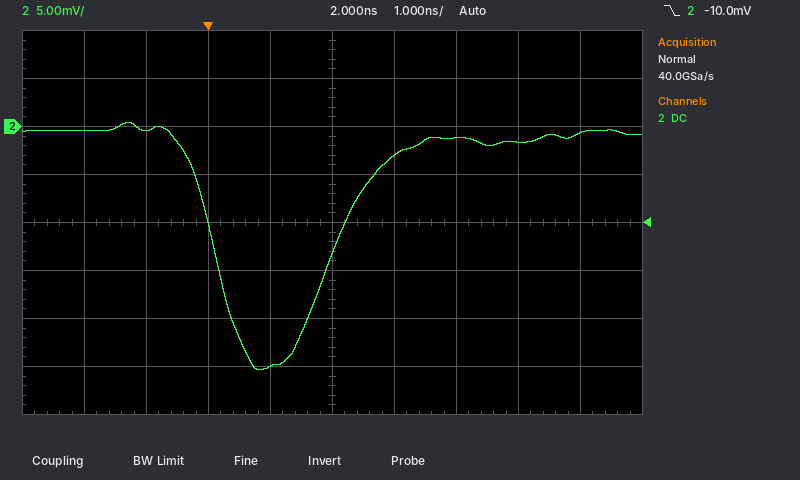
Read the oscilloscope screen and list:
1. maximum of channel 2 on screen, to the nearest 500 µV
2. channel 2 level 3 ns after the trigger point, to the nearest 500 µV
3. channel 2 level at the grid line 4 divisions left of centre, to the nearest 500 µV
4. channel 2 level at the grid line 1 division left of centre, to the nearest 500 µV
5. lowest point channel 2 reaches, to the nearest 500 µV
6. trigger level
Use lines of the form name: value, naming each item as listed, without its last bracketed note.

maximum of channel 2 on screen, to the nearest 500 µV: 500 µV
channel 2 level 3 ns after the trigger point, to the nearest 500 µV: -3.0 mV
channel 2 level at the grid line 4 divisions left of centre, to the nearest 500 µV: -500 µV
channel 2 level at the grid line 1 division left of centre, to the nearest 500 µV: -25.0 mV
lowest point channel 2 reaches, to the nearest 500 µV: -25.5 mV
trigger level: -10.0 mV
